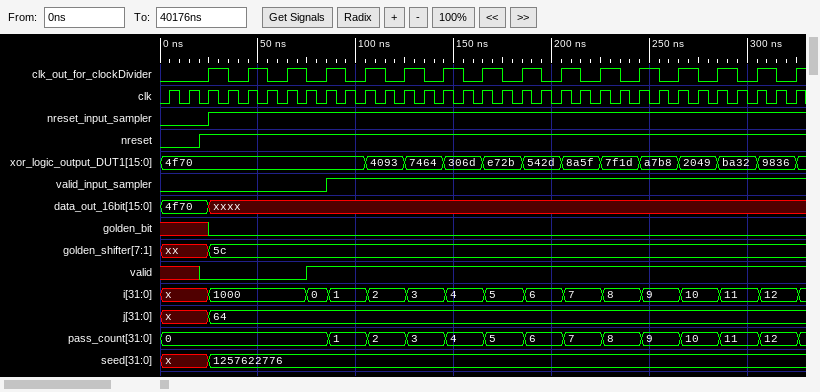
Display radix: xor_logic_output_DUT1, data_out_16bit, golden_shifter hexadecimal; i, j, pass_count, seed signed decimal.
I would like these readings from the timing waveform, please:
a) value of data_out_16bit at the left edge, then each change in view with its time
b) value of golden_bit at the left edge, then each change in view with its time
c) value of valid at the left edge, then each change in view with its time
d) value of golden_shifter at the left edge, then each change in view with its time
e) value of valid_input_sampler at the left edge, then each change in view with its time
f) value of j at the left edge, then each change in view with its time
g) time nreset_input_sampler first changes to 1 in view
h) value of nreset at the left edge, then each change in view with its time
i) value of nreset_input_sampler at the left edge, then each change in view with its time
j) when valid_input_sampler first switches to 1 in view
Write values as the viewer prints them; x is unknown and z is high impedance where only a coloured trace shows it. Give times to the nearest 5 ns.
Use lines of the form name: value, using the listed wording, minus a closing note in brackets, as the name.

value of data_out_16bit at the left edge, then each change in view with its time: 4f70, xxxx at 25 ns
value of golden_bit at the left edge, then each change in view with its time: x, 0 at 25 ns
value of valid at the left edge, then each change in view with its time: x, 0 at 20 ns, 1 at 75 ns
value of golden_shifter at the left edge, then each change in view with its time: xx, 5c at 25 ns
value of valid_input_sampler at the left edge, then each change in view with its time: 0, 1 at 85 ns
value of j at the left edge, then each change in view with its time: x, 64 at 25 ns
time nreset_input_sampler first changes to 1 in view: 25 ns
value of nreset at the left edge, then each change in view with its time: 0, 1 at 20 ns
value of nreset_input_sampler at the left edge, then each change in view with its time: 0, 1 at 25 ns
when valid_input_sampler first switches to 1 in view: 85 ns
